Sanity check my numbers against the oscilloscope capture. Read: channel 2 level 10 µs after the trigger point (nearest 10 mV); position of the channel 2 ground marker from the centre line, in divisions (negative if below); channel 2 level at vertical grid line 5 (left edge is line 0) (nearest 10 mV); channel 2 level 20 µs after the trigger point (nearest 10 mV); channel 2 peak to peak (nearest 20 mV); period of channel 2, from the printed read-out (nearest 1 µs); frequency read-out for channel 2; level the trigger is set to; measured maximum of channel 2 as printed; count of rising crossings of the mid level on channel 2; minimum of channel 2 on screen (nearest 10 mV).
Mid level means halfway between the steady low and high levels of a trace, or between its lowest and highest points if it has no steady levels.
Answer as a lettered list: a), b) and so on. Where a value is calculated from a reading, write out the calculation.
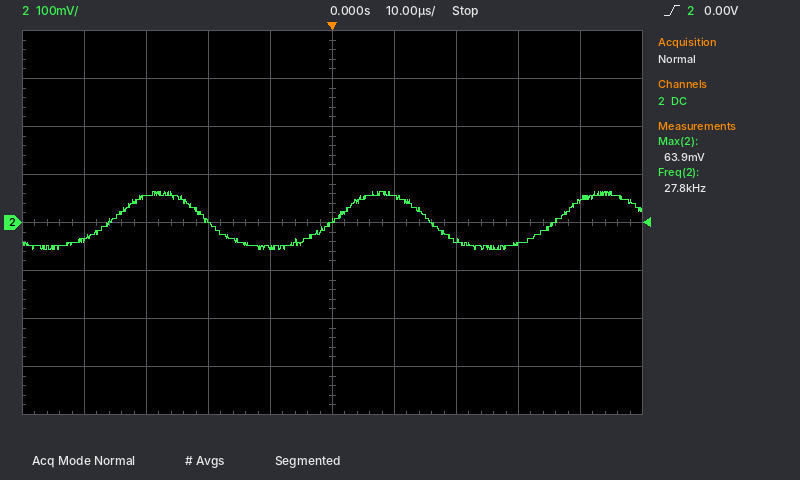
a) 50 mV
b) 0.0 div
c) 0 mV
d) -40 mV
e) 120 mV
f) 1 / 27.8 kHz ≈ 36 µs
g) 27.8 kHz
h) 0.00 V
i) 63.9 mV
j) 3
k) -60 mV
